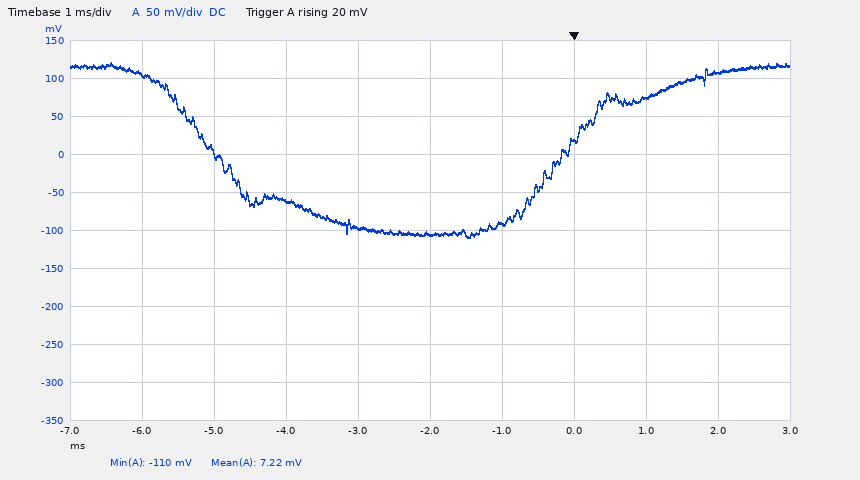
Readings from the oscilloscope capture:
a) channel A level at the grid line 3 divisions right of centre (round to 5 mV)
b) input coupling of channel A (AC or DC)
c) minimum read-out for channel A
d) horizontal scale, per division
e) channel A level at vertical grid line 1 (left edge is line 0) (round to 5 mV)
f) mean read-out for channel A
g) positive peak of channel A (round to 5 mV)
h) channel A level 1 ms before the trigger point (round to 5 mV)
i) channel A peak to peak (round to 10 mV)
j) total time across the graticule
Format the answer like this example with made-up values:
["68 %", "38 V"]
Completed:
["75 mV", "DC", "-110 mV", "1 ms", "105 mV", "7.22 mV", "120 mV", "-90 mV", "230 mV", "10 ms"]
